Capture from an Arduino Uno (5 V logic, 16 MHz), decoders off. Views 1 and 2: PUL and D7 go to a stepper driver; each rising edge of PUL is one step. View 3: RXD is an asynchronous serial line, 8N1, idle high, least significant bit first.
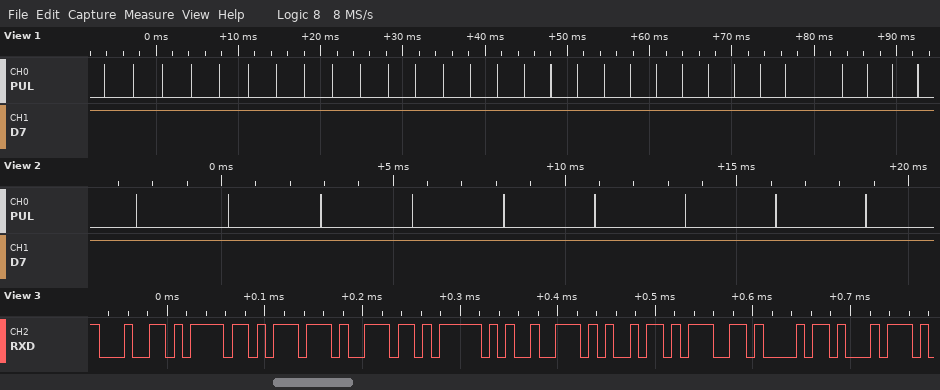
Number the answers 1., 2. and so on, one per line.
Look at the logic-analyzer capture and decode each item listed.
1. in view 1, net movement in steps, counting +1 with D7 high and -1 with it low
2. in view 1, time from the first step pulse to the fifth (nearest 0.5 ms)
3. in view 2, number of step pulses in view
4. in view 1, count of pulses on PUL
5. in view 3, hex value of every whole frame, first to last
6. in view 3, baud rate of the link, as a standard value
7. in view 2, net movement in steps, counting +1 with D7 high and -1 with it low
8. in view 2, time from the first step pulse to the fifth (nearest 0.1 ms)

1. +30
2. 14.0 ms
3. 9
4. 30
5. 0x64 0x6F 0x77 0x6E 0x5F 0x72 0x69 0x67 0x68 0x74
6. 115200 baud
7. +9
8. 10.7 ms
